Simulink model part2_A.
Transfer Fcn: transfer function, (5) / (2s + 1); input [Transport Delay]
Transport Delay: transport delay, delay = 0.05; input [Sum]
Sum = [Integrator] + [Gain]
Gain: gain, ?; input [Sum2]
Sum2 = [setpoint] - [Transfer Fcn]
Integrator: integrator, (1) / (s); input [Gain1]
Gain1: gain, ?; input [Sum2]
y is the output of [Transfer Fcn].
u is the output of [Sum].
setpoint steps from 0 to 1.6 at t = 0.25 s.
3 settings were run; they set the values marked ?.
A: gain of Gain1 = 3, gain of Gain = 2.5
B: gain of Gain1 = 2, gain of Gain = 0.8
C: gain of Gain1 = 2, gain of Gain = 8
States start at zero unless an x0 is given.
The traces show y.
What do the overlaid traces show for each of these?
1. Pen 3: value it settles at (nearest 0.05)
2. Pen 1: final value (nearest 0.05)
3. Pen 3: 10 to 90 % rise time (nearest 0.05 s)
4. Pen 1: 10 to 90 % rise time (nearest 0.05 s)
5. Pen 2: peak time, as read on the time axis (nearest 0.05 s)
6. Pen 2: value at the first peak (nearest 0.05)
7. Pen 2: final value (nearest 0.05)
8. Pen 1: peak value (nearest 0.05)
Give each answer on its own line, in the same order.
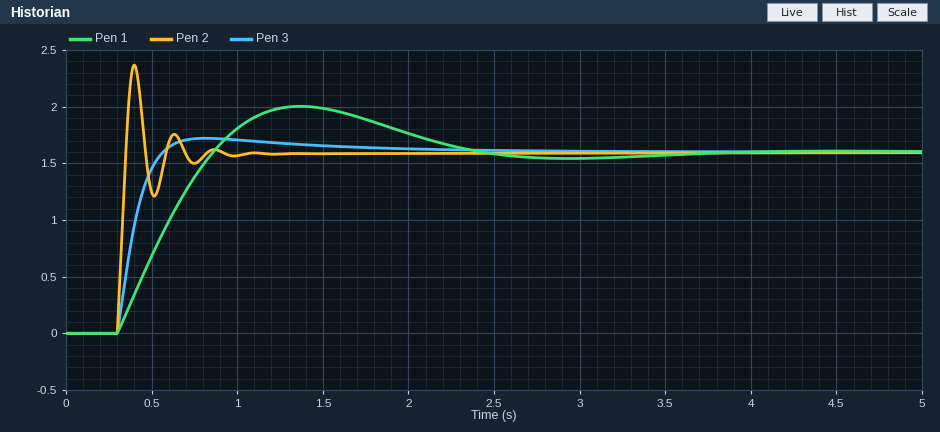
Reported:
1.60
1.60
0.20 s
0.45 s
0.40 s
2.35
1.60
2.00
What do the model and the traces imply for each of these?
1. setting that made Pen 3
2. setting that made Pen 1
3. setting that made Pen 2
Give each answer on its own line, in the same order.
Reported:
A
B
C
